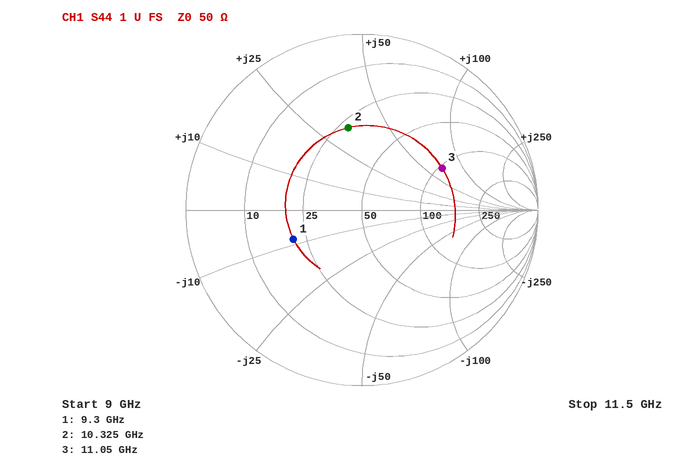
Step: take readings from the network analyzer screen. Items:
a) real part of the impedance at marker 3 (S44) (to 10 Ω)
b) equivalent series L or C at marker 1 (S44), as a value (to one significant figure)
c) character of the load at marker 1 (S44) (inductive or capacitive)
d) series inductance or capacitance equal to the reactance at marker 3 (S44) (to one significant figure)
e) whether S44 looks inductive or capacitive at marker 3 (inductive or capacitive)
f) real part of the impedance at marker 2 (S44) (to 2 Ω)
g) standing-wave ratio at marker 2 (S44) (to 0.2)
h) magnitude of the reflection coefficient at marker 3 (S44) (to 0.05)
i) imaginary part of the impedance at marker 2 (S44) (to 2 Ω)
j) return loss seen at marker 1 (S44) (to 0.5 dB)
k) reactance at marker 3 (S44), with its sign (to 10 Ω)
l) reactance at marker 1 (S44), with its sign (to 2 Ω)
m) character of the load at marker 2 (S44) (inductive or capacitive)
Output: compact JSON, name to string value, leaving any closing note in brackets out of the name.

{"real part of the impedance at marker 3 (S44)": "100 Ω", "equivalent series L or C at marker 1 (S44), as a value": "2 pF", "character of the load at marker 1 (S44)": "capacitive", "series inductance or capacitance equal to the reactance at marker 3 (S44)": "1.0 nH", "whether S44 looks inductive or capacitive at marker 3": "inductive", "real part of the impedance at marker 2 (S44)": "28 Ω", "standing-wave ratio at marker 2 (S44)": "2.8", "magnitude of the reflection coefficient at marker 3 (S44)": "0.50", "imaginary part of the impedance at marker 2 (S44)": "+34 Ω", "return loss seen at marker 1 (S44)": "7.5 dB", "reactance at marker 3 (S44), with its sign": "+70 Ω", "reactance at marker 1 (S44), with its sign": "-8 Ω", "character of the load at marker 2 (S44)": "inductive"}
